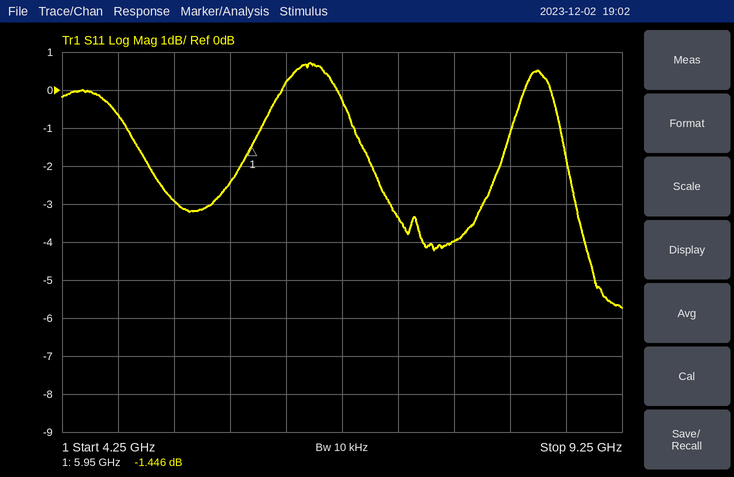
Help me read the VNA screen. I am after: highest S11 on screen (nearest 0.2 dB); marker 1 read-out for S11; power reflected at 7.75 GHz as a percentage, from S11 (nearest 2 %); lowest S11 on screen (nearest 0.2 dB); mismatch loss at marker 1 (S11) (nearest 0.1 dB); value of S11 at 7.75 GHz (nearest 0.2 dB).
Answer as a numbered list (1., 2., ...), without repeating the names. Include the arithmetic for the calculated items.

1. 0.8 dB
2. -1.446 dB
3. 10^(-4/10) ≈ 40 %
4. -5.8 dB
5. −10 log10(1 − 10^(-1.446/10)) ≈ 5.5 dB
6. -4.0 dB
